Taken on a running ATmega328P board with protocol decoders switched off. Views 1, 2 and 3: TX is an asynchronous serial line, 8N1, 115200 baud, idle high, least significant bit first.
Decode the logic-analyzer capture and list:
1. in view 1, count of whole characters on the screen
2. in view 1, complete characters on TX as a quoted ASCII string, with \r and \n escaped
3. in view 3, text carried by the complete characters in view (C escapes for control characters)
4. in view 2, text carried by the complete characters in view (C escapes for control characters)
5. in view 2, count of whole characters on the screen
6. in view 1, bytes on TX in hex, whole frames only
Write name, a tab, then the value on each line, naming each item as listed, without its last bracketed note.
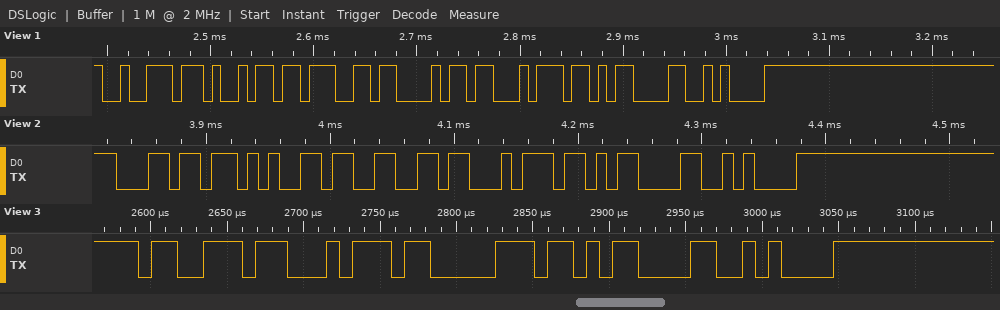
in view 1, count of whole characters on the screen	7
in view 1, complete characters on TX as a quoted ASCII string, with \r and \n escaped	"right\r\n"
in view 3, text carried by the complete characters in view	"stp\r\n"
in view 2, text carried by the complete characters in view	"left\r\n"
in view 2, count of whole characters on the screen	6
in view 1, bytes on TX in hex, whole frames only	0x72 0x69 0x67 0x68 0x74 0x0D 0x0A
